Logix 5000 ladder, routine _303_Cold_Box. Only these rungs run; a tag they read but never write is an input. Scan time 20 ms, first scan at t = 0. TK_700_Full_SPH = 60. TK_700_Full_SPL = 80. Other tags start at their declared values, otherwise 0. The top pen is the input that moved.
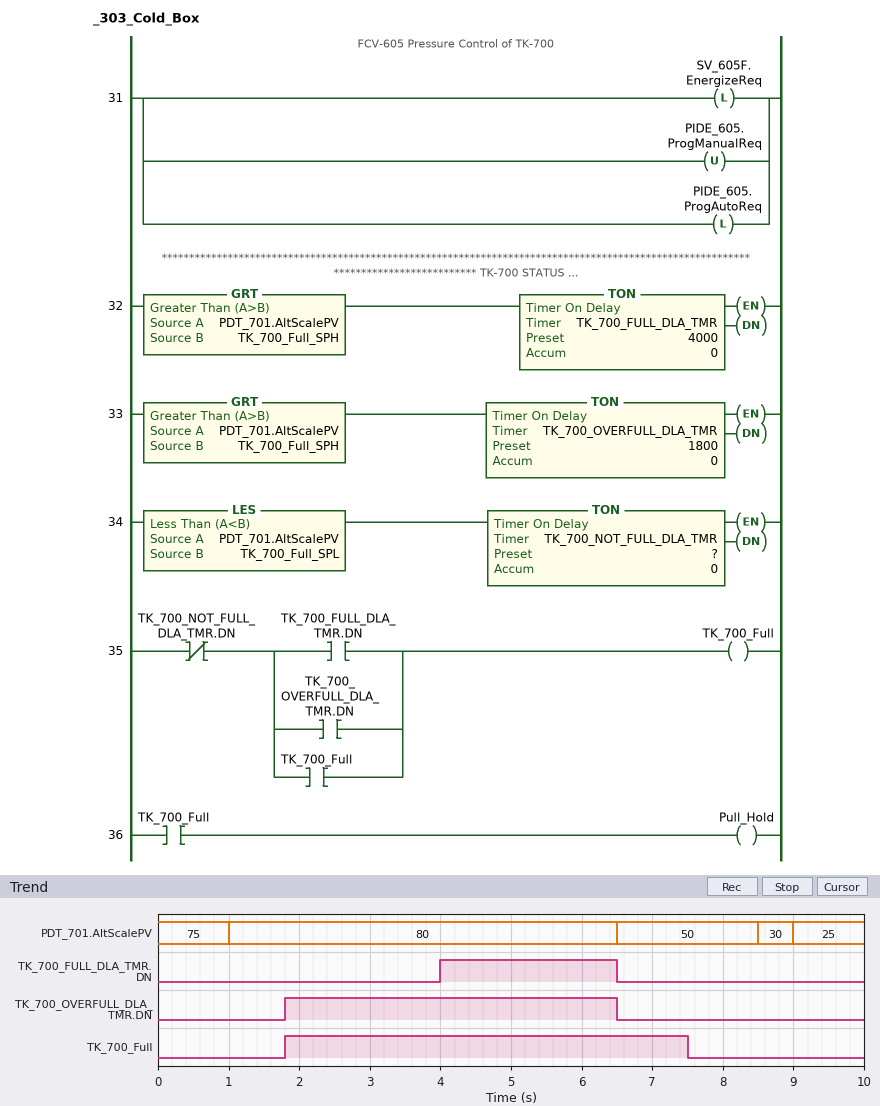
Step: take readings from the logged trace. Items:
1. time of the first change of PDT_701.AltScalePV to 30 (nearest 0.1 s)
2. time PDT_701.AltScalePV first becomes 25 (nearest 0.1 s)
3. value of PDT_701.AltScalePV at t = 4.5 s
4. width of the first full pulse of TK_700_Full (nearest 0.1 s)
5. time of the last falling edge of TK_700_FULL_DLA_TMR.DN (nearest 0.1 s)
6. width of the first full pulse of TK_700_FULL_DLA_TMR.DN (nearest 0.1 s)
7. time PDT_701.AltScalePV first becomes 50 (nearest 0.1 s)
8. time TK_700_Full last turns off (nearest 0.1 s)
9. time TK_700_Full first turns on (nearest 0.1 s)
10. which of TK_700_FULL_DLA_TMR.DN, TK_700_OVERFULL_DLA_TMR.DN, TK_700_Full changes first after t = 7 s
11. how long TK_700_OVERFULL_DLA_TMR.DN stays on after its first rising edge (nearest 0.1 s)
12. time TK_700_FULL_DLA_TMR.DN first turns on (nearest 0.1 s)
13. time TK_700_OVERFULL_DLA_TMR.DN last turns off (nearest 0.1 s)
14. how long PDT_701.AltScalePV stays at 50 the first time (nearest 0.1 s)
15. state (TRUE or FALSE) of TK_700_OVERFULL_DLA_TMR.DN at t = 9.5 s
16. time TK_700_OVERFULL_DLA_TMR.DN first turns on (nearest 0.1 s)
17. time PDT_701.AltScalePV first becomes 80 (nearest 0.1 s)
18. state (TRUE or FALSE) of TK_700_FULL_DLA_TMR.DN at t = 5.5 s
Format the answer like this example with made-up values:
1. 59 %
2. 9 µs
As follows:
1. 8.5 s
2. 9.0 s
3. 80
4. 5.7 s
5. 6.5 s
6. 2.5 s
7. 6.5 s
8. 7.5 s
9. 1.8 s
10. TK_700_Full
11. 4.7 s
12. 4.0 s
13. 6.5 s
14. 2.0 s
15. FALSE
16. 1.8 s
17. 1.0 s
18. TRUE
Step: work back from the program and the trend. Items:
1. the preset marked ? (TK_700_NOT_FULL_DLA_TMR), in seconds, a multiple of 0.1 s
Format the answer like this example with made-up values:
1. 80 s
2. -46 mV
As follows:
1. 1.0 s
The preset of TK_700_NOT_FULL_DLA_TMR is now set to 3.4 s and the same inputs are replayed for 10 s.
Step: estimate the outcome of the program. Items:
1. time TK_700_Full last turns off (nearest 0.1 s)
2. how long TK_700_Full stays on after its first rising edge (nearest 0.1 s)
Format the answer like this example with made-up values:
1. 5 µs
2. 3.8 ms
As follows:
1. 9.9 s
2. 8.1 s
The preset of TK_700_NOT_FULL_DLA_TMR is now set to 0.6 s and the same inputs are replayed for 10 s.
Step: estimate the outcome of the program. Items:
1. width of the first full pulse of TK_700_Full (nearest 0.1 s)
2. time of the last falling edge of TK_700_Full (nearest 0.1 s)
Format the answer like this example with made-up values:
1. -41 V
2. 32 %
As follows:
1. 5.3 s
2. 7.1 s
